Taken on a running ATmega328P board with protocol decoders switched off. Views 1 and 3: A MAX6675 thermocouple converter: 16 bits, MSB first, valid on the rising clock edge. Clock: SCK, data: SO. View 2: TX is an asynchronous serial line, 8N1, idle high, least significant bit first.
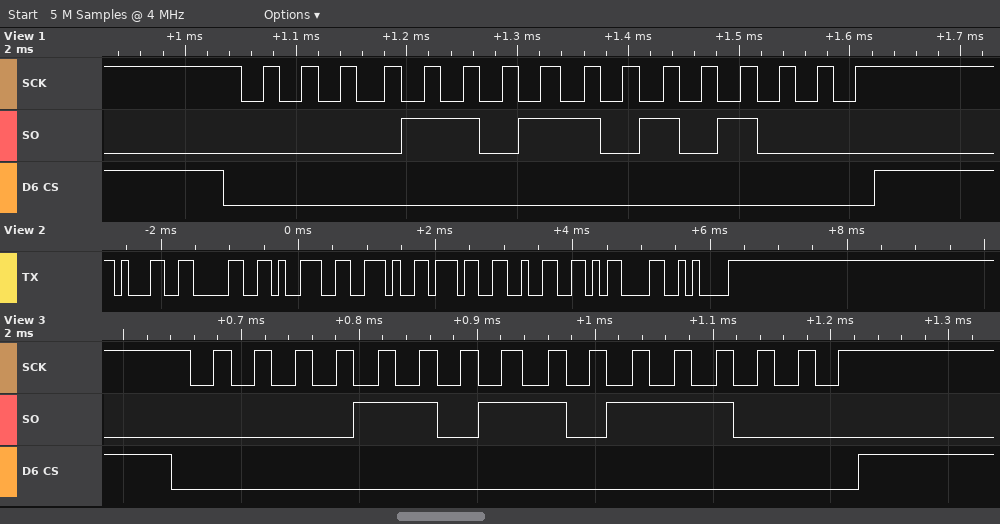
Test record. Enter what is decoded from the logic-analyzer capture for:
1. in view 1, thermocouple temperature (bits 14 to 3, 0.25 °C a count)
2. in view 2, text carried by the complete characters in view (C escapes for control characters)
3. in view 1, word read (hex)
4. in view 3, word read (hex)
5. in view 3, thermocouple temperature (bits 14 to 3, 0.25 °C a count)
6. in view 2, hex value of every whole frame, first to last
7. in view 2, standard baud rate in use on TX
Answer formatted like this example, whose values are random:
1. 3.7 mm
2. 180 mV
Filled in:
1. 109.25 °C
2. "109.72\r\n"
3. 0x0DA8
4. 0x0DB8
5. 109.75 °C
6. 0x31 0x30 0x39 0x2E 0x37 0x32 0x0D 0x0A
7. 9600 baud
